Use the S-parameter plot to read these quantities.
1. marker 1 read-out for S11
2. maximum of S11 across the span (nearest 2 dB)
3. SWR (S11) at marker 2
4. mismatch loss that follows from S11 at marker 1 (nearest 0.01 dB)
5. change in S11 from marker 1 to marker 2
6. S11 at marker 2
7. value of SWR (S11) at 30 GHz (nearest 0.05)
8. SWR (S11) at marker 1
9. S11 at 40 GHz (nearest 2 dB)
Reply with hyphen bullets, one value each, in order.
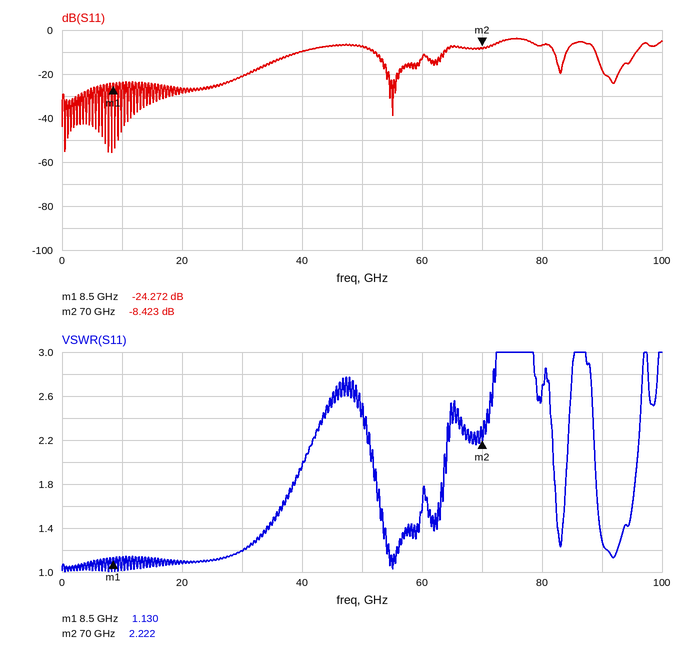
- -24.272 dB
- -4 dB
- 2.222
- 0.02 dB
- 15.849 dB
- -8.423 dB
- 1.20
- 1.130
- -10 dB
